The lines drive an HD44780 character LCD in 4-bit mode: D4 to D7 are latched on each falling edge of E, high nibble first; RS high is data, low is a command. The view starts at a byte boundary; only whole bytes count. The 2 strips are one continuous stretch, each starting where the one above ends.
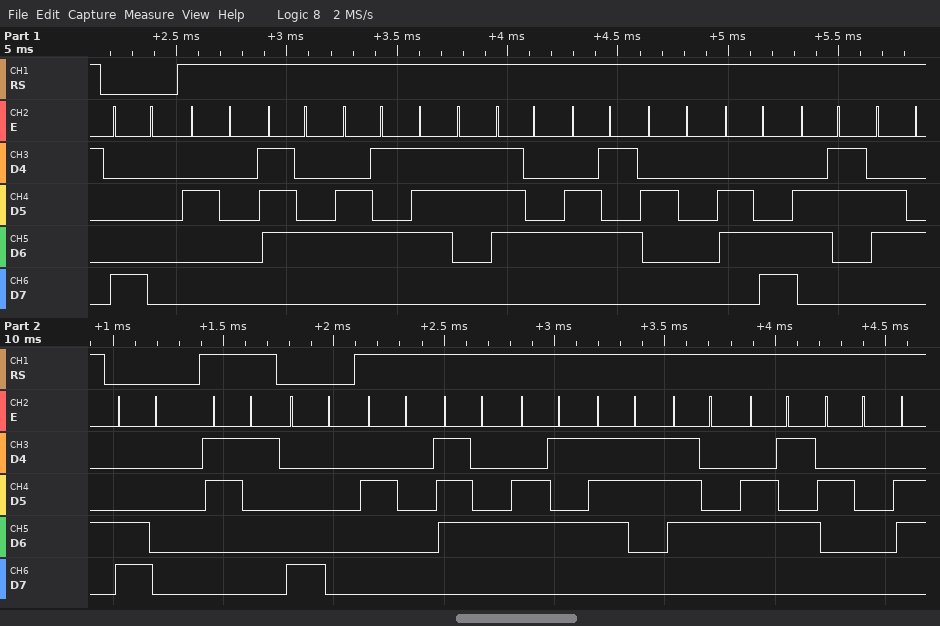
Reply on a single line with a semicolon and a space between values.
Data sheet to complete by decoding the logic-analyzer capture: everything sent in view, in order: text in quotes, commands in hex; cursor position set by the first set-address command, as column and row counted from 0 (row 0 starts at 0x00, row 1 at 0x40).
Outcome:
0x80 " teste lcd" 0xC0 "1" 0x80 " teste "; column 0, row 0
